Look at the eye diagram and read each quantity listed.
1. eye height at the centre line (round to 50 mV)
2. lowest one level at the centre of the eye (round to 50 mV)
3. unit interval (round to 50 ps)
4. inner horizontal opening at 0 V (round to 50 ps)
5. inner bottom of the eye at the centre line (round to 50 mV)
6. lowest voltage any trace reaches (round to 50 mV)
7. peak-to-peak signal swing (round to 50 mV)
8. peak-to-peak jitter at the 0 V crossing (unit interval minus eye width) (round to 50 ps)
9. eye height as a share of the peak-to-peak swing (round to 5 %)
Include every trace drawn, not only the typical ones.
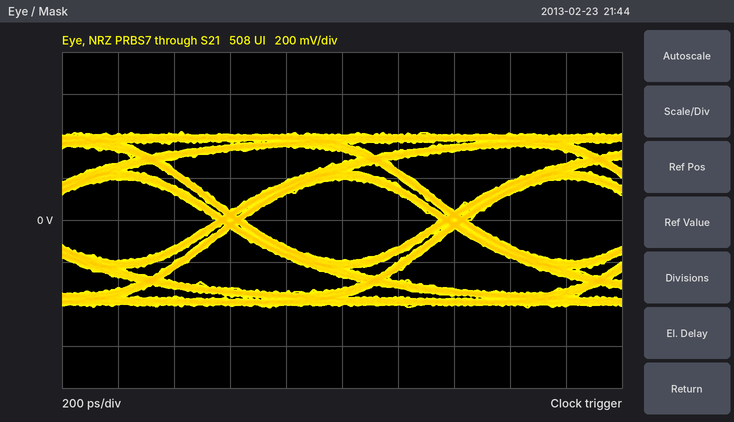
400 mV
200 mV
800 ps
700 ps
-200 mV
-400 mV
850 mV
100 ps
45 %
